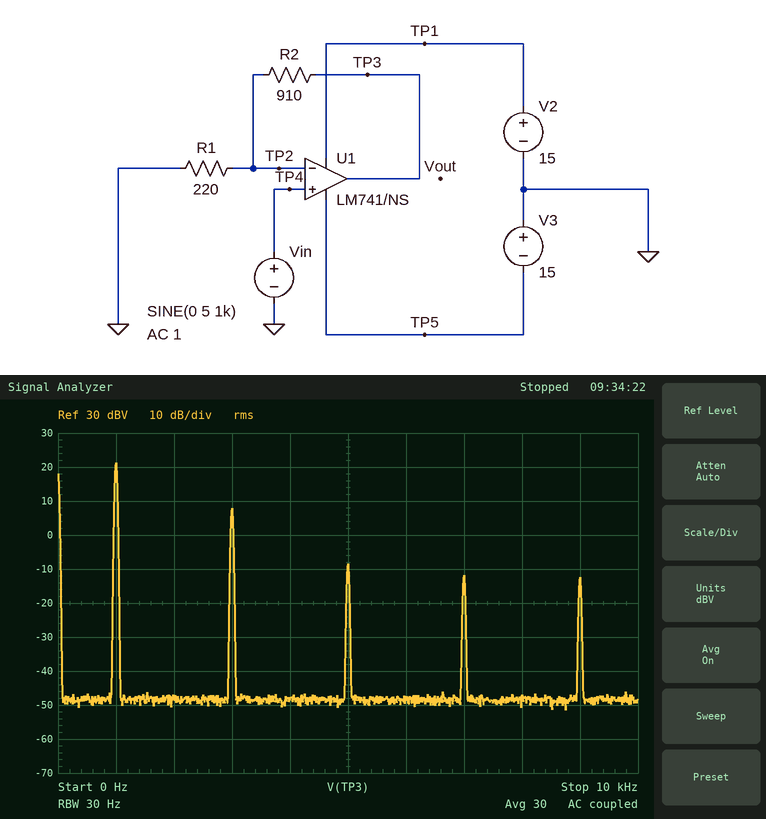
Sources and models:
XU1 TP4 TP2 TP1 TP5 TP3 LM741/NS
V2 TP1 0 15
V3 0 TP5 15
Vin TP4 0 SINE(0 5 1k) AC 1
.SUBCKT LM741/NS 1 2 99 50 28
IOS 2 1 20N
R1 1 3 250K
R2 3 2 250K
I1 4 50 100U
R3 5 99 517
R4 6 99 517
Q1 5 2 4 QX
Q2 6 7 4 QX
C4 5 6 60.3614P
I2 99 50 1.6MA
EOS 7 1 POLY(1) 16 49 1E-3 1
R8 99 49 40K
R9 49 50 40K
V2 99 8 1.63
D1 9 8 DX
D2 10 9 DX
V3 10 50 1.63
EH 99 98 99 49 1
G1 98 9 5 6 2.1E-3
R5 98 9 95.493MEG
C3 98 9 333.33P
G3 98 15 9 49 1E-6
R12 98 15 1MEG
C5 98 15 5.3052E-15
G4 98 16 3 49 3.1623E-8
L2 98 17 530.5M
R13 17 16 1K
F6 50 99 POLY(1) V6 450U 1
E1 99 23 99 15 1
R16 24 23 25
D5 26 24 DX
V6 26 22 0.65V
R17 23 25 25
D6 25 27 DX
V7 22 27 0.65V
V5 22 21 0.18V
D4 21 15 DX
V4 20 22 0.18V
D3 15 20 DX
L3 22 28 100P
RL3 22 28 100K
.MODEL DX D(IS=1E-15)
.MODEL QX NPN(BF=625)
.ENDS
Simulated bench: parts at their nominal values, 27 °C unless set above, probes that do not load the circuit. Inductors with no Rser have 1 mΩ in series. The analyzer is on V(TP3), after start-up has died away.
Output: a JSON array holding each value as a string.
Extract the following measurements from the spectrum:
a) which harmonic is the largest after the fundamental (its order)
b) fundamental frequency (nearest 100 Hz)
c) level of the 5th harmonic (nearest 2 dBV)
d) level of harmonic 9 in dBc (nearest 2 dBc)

["3", "1.0 kHz", "-8 dBV", "-34 dBc"]
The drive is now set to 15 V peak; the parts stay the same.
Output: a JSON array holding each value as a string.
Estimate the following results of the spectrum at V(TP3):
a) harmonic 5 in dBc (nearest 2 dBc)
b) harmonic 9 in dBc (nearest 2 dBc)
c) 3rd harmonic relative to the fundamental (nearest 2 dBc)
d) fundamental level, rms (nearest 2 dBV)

["-16 dBc", "-30 dBc", "-10 dBc", "22 dBV"]
